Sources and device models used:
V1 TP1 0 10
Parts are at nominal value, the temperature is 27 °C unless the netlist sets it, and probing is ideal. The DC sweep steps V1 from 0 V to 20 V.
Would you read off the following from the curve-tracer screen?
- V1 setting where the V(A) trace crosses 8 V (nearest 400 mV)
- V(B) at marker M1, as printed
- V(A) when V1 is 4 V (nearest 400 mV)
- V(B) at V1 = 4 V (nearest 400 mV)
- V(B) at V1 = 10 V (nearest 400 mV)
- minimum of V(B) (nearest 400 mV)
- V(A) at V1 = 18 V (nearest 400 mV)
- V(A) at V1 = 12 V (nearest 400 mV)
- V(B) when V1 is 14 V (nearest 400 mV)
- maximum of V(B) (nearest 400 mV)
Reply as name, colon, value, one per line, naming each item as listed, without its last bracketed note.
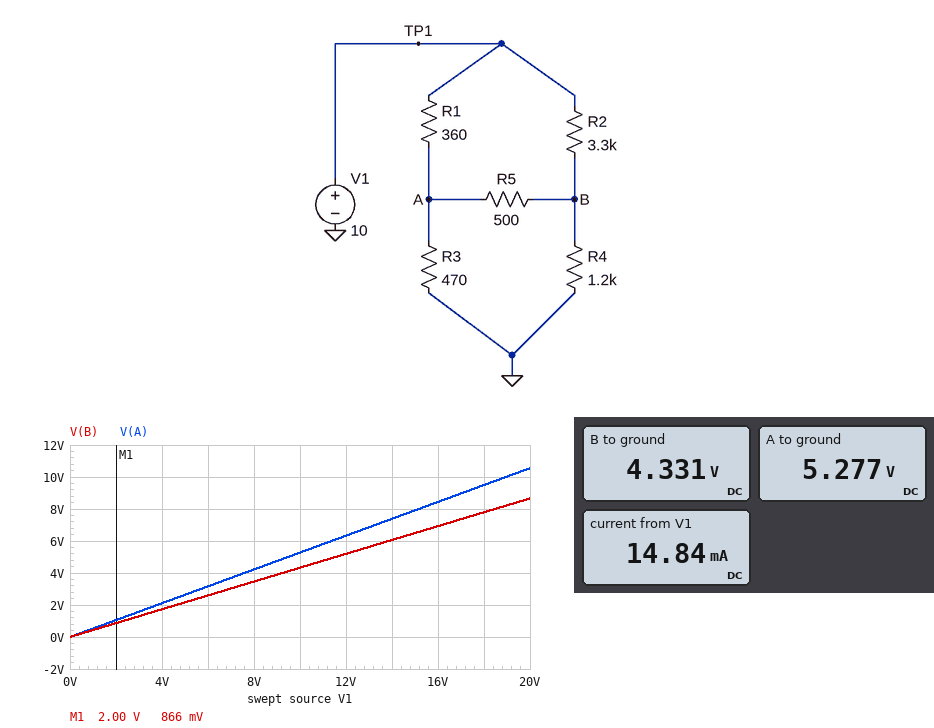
V1 setting where the V(A) trace crosses 8 V: 15.2 V
V(B) at marker M1, as printed: 866 mV
V(A) when V1 is 4 V: 2.0 V
V(B) at V1 = 4 V: 1.6 V
V(B) at V1 = 10 V: 4.4 V
minimum of V(B): 0 V
V(A) at V1 = 18 V: 9.6 V
V(A) at V1 = 12 V: 6.4 V
V(B) when V1 is 14 V: 6.0 V
maximum of V(B): 8.8 V
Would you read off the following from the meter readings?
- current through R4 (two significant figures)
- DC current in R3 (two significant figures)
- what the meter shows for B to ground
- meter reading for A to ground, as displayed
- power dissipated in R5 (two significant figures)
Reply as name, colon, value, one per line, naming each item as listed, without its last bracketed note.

current through R4: 3.6 mA
DC current in R3: 11 mA
what the meter shows for B to ground: 4.331 V
meter reading for A to ground, as displayed: 5.277 V
power dissipated in R5: 1.8 mW
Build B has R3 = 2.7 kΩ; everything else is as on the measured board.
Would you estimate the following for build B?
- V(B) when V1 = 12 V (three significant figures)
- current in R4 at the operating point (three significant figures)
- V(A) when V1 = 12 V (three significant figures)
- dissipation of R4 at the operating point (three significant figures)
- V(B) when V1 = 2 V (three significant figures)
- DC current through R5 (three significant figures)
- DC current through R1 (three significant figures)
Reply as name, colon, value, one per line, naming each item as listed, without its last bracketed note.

V(B) when V1 = 12 V: 7.03 V
current in R4 at the operating point: 4.88 mA
V(A) when V1 = 12 V: 9.21 V
dissipation of R4 at the operating point: 28.6 mW
V(B) when V1 = 2 V: 1.17 V
DC current through R5: 3.63 mA
DC current through R1: 6.47 mA
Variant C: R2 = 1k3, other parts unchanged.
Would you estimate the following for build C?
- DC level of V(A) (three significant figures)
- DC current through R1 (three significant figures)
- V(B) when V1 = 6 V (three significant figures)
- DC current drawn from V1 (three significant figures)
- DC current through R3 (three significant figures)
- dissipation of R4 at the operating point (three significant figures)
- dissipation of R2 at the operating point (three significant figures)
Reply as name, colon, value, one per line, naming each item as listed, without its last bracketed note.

DC level of V(A): 5.53 V
DC current through R1: 12.4 mA
V(B) when V1 = 6 V: 3.12 V
DC current drawn from V1: 16.1 mA
DC current through R3: 11.8 mA
dissipation of R4 at the operating point: 22.6 mW
dissipation of R2 at the operating point: 17.7 mW
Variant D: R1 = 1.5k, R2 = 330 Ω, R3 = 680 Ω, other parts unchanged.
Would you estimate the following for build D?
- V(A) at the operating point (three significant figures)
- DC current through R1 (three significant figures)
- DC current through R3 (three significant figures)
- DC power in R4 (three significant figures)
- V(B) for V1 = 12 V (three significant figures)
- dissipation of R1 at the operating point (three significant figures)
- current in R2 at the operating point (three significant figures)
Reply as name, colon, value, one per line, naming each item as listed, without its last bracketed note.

V(A) at the operating point: 4.92 V
DC current through R1: 3.39 mA
DC current through R3: 7.24 mA
DC power in R4: 39.1 mW
V(B) for V1 = 12 V: 8.22 V
dissipation of R1 at the operating point: 17.2 mW
current in R2 at the operating point: 9.56 mA
